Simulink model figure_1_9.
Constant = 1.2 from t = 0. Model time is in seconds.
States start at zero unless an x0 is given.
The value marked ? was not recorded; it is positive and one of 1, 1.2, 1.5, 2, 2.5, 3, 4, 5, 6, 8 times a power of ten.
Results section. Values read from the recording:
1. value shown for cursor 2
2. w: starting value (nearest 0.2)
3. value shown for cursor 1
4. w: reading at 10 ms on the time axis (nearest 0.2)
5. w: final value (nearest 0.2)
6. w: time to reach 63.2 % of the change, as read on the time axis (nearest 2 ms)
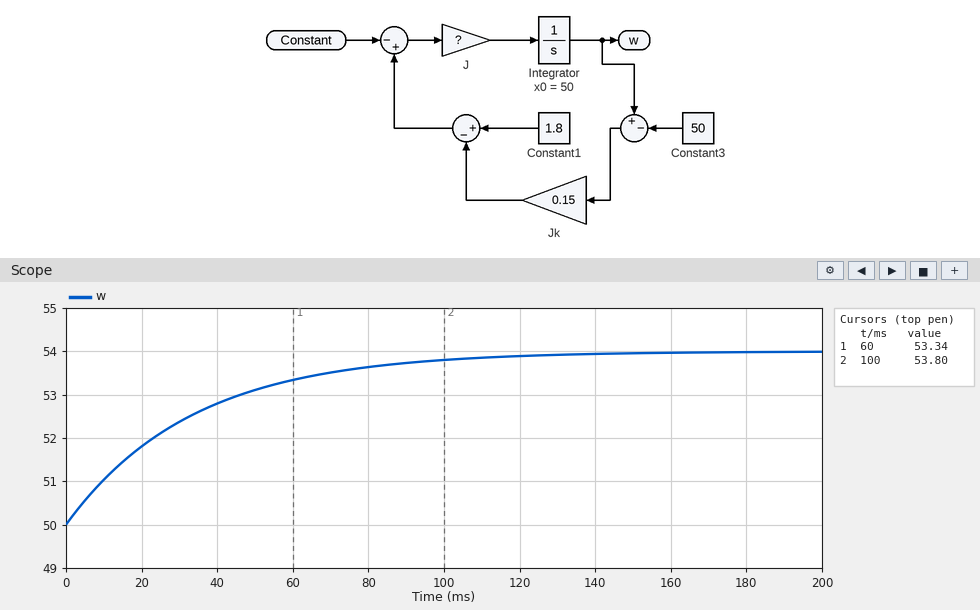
53.80
50.0
53.34
51.0
54.0
34 ms
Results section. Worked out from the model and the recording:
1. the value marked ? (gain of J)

200
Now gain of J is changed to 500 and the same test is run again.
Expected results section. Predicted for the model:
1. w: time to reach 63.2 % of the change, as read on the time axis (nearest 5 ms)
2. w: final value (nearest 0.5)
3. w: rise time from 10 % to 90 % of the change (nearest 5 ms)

15 ms
54.0
30 ms
